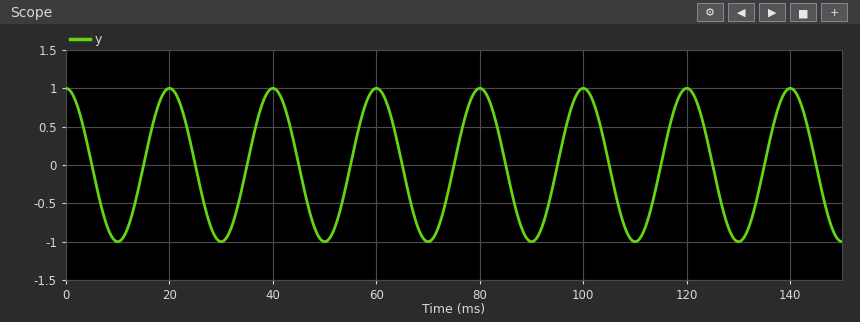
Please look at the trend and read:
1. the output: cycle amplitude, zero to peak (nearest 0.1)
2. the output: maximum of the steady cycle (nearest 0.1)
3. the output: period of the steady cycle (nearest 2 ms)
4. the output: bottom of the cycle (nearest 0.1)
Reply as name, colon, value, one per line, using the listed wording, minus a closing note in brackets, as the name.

the output: cycle amplitude, zero to peak: 1.0
the output: maximum of the steady cycle: 1.0
the output: period of the steady cycle: 20 ms
the output: bottom of the cycle: -1.0
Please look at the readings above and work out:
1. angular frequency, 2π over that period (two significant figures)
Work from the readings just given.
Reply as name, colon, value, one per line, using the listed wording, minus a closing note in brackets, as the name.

angular frequency, 2π over that period: 0.31 rad/ms
